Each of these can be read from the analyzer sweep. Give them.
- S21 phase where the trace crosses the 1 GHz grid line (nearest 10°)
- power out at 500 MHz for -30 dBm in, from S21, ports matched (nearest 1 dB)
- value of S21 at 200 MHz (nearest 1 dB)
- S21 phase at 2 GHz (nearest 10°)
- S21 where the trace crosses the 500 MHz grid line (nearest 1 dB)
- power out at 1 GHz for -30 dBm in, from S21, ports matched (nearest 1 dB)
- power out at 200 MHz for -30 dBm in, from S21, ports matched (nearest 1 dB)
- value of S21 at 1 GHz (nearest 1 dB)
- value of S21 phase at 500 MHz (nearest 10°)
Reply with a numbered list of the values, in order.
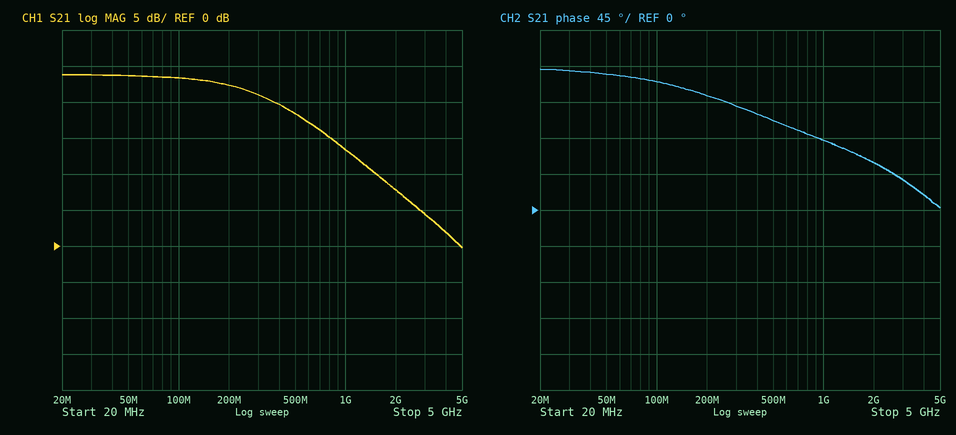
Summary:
1. 90°
2. -12 dBm
3. 22 dB
4. 60°
5. 18 dB
6. -17 dBm
7. -8 dBm
8. 13 dB
9. 110°
